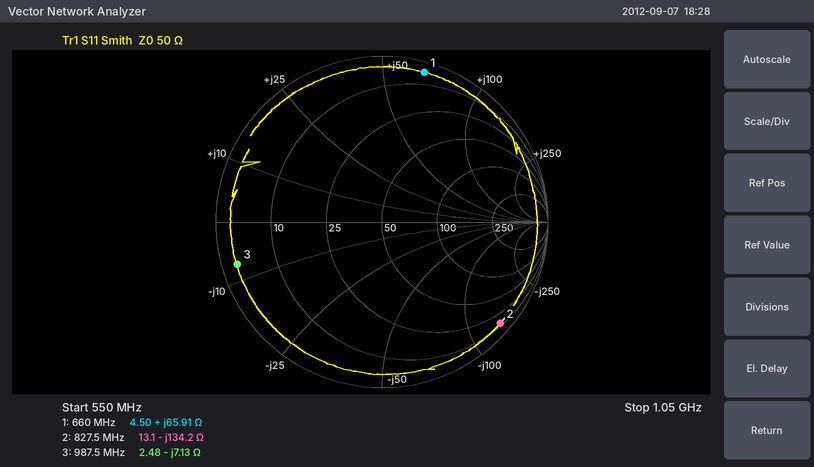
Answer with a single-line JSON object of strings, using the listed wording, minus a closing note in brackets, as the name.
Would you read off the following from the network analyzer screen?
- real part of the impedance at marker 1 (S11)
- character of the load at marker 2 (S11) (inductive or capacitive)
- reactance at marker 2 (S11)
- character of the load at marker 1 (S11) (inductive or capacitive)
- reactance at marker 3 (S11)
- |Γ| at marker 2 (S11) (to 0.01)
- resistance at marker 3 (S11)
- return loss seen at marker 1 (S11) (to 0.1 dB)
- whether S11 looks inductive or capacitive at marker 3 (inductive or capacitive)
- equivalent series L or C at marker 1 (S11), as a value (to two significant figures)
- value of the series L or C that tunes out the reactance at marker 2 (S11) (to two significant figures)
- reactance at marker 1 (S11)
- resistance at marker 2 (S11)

{"real part of the impedance at marker 1": "4.50 Ω", "character of the load at marker 2 (S11)": "capacitive", "reactance at marker 2": "-134.2 Ω", "character of the load at marker 1 (S11)": "inductive", "reactance at marker 3": "-7.13 Ω", "|Γ| at marker 2 (S11)": "0.94", "resistance at marker 3": "2.48 Ω", "return loss seen at marker 1 (S11)": "0.6 dB", "whether S11 looks inductive or capacitive at marker 3": "capacitive", "equivalent series L or C at marker 1 (S11), as a value": "16 nH", "value of the series L or C that tunes out the reactance at marker 2 (S11)": "26 nH", "reactance at marker 1": "+65.91 Ω", "resistance at marker 2": "13.1 Ω"}
